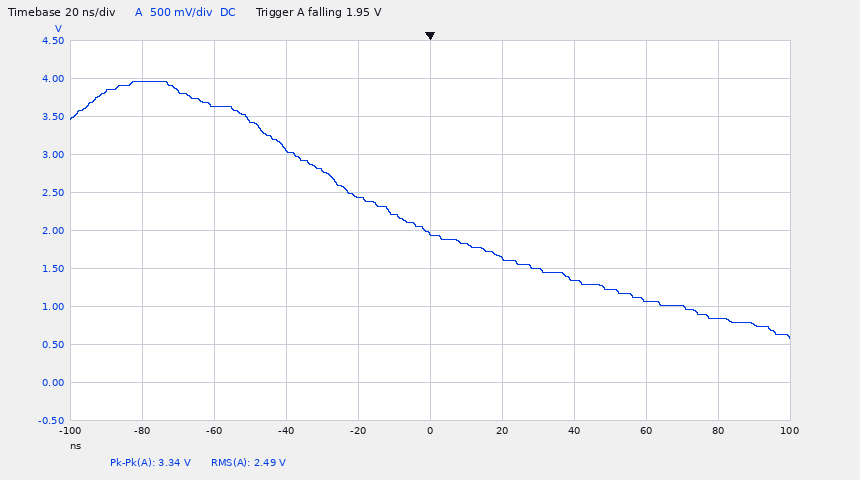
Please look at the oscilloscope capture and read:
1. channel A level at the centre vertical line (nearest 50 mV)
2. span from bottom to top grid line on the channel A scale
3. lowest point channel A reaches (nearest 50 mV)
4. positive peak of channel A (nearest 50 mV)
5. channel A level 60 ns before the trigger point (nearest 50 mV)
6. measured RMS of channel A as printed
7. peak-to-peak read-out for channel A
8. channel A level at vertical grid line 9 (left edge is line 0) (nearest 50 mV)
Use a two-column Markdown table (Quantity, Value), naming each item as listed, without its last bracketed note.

| Quantity | Value |
|---|---|
| channel A level at the centre vertical line | 1.95 V |
| span from bottom to top grid line on the channel A scale | 5 V |
| lowest point channel A reaches | 600 mV |
| positive peak of channel A | 3.95 V |
| channel A level 60 ns before the trigger point | 3.65 V |
| measured RMS of channel A as printed | 2.49 V |
| peak-to-peak read-out for channel A | 3.34 V |
| channel A level at vertical grid line 9 (left edge is line 0) | 850 mV |
